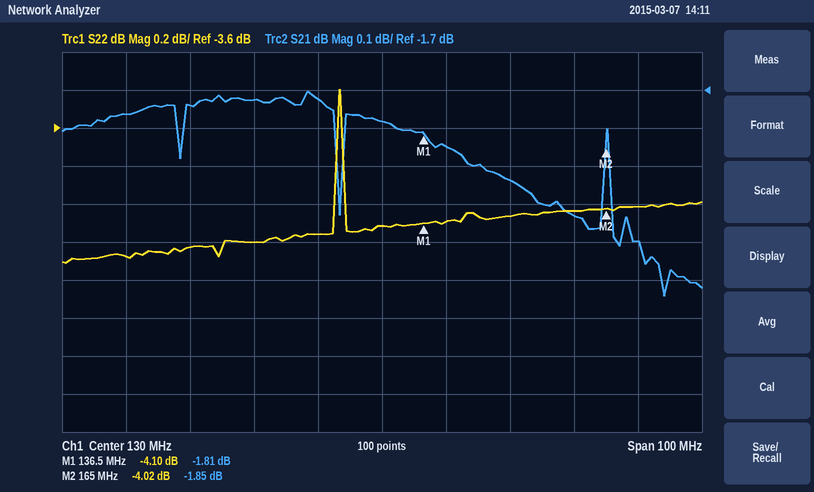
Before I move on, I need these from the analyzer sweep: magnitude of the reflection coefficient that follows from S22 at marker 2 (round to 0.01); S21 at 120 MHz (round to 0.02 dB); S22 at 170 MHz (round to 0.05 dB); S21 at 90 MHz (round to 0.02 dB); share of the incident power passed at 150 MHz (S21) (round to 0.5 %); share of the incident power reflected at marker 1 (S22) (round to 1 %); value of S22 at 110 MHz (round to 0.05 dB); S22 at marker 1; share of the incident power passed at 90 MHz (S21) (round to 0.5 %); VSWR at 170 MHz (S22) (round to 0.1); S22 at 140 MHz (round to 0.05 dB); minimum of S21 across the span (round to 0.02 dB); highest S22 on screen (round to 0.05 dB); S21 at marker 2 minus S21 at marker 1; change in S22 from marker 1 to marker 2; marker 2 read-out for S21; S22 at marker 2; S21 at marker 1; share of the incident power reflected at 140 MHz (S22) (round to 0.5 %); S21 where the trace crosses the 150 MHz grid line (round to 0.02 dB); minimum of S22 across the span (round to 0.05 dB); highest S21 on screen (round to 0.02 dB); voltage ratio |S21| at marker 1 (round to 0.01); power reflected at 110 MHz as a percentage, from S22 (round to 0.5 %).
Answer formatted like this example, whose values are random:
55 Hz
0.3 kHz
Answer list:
0.63
-1.72 dB
-4.00 dB
-1.76 dB
64.0 %
39 %
-4.20 dB
-4.10 dB
66.5 %
4.4
-4.10 dB
-2.24 dB
-3.40 dB
-0.04 dB
0.08 dB
-1.85 dB
-4.02 dB
-1.81 dB
39.0 %
-1.94 dB
-4.30 dB
-1.70 dB
0.81
38.0 %
